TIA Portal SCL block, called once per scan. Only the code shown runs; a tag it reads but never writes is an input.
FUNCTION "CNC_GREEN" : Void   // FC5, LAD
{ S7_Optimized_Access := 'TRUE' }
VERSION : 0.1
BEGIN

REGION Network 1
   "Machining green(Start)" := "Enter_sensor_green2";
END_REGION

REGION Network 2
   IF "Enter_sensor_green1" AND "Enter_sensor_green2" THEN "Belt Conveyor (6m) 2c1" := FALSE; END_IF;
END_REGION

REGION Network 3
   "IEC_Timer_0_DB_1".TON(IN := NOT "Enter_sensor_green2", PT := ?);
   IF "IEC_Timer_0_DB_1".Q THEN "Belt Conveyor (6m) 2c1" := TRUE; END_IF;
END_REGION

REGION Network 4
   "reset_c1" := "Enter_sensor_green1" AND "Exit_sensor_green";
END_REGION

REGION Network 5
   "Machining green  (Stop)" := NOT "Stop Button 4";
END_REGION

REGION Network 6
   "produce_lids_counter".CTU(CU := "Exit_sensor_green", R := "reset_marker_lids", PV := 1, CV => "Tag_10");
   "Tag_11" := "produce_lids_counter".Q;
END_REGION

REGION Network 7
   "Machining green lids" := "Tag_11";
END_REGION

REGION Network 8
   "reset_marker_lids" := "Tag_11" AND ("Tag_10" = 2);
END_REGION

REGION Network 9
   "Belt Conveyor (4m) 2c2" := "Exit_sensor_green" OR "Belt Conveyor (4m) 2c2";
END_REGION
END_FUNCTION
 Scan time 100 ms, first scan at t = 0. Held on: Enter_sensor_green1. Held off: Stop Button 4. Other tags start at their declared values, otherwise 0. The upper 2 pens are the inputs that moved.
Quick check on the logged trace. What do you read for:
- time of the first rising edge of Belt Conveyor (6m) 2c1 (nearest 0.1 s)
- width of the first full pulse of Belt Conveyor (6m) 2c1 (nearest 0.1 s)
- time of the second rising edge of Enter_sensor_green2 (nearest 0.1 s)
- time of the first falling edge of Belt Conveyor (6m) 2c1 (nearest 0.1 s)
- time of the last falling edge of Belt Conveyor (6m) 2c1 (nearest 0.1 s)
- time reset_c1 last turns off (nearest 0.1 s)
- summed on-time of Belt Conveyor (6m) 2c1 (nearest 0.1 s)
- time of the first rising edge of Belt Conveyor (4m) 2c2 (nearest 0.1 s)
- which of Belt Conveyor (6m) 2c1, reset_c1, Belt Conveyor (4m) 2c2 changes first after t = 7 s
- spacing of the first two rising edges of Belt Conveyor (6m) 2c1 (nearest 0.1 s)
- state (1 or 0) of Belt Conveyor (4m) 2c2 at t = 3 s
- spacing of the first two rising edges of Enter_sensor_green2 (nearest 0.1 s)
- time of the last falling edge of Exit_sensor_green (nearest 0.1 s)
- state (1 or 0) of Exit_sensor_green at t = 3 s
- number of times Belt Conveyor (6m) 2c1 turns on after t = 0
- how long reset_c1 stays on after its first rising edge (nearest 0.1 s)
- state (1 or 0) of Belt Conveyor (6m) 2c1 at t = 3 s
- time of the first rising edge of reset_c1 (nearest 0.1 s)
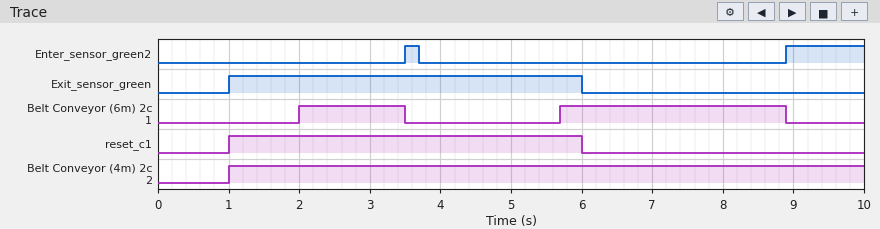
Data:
2.0 s
1.5 s
8.9 s
3.5 s
8.9 s
6.0 s
4.7 s
1.0 s
Belt Conveyor (6m) 2c1
3.7 s
1
5.4 s
6.0 s
1
2
5.0 s
1
1.0 s
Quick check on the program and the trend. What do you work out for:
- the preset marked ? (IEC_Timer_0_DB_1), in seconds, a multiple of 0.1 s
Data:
2.0 s
